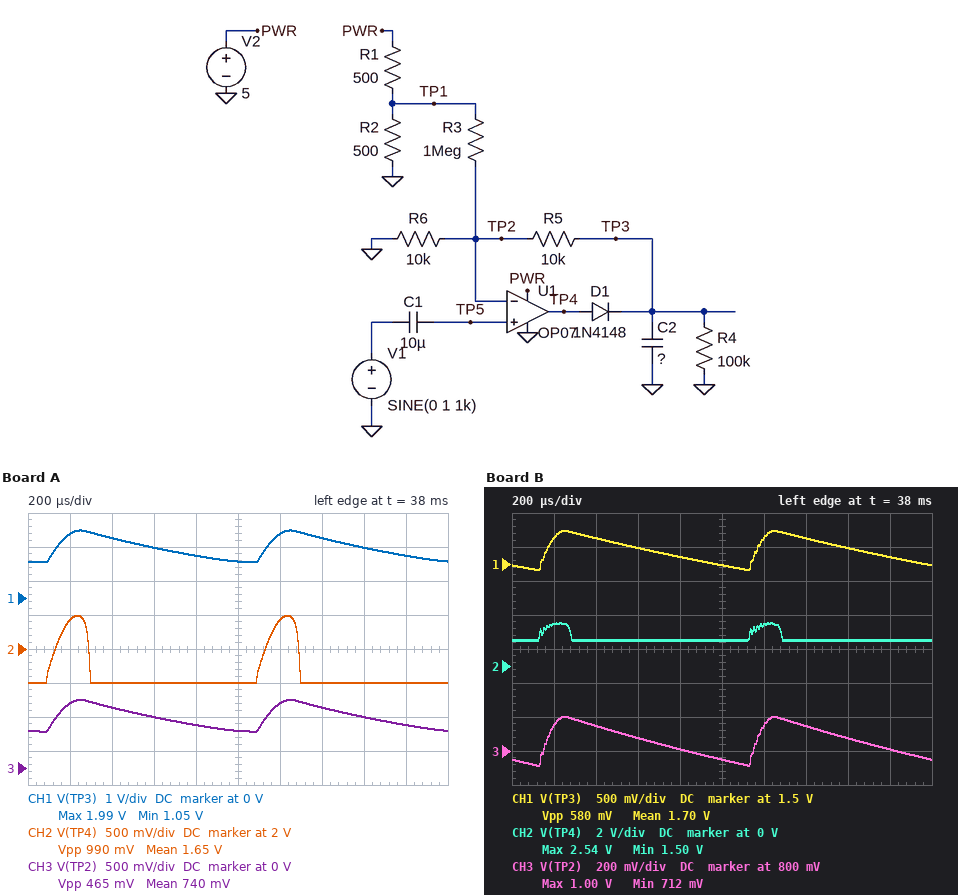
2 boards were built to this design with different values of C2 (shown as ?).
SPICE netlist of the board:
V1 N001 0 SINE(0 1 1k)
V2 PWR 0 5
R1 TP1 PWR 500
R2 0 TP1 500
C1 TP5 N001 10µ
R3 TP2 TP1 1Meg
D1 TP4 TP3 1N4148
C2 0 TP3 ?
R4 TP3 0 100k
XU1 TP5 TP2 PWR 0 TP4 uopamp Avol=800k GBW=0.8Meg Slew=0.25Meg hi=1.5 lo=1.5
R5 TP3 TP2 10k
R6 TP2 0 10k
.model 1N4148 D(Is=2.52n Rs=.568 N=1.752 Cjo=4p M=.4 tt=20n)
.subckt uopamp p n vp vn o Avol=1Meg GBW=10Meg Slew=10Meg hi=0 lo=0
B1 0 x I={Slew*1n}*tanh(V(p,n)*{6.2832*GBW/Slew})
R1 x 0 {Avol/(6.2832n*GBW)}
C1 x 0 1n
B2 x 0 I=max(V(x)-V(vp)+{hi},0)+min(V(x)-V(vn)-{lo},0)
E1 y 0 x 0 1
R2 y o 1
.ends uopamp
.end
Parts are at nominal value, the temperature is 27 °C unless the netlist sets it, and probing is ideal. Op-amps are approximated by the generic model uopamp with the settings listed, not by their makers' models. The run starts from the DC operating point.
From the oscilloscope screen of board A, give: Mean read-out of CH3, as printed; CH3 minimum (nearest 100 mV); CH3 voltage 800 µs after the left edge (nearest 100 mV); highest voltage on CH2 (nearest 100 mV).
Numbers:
740 mV
500 mV
600 mV
2.5 V
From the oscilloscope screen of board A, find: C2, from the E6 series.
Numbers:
68 nF
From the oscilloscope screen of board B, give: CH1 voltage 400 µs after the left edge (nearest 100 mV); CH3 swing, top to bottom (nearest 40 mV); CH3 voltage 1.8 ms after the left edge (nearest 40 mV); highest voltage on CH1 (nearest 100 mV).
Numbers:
1.9 V
280 mV
800 mV
2.0 V
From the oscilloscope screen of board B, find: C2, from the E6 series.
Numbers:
150 nF
